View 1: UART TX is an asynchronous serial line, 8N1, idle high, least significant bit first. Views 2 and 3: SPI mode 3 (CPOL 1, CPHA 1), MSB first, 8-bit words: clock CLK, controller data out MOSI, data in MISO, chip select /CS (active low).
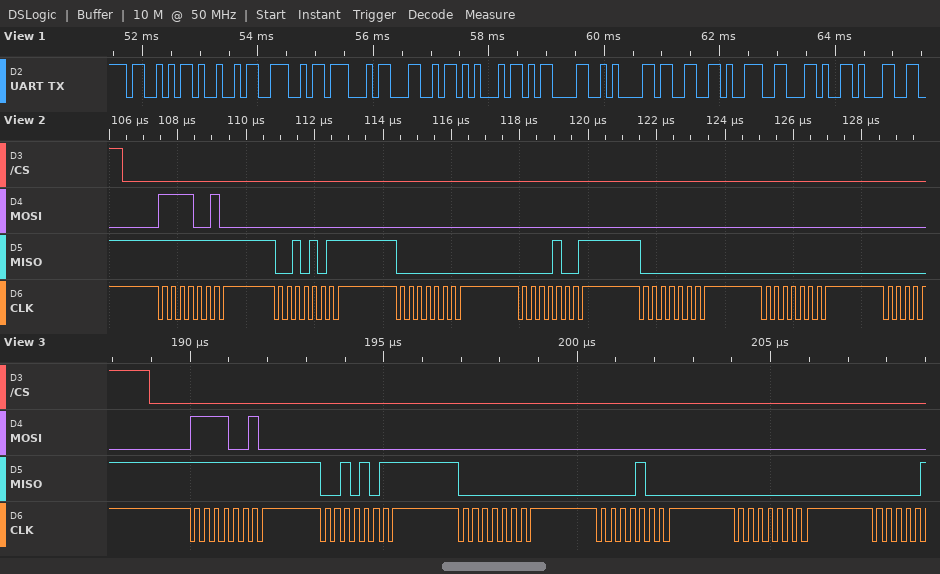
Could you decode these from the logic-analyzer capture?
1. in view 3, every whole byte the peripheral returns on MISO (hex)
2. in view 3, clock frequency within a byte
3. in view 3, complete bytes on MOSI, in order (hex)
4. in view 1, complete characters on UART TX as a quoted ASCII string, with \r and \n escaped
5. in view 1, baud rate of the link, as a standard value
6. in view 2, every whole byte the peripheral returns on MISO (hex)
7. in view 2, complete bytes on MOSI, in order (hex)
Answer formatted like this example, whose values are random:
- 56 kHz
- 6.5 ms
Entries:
- 0xFF 0x2B 0x00 0x08 0x00
- 4 MHz
- 0xF2 0x00 0x00 0x00 0x00
- "SINGLE\r\n39,1"
- 9600 baud
- FF 2B 00 09 00 00
- F2 00 00 00 00 00
